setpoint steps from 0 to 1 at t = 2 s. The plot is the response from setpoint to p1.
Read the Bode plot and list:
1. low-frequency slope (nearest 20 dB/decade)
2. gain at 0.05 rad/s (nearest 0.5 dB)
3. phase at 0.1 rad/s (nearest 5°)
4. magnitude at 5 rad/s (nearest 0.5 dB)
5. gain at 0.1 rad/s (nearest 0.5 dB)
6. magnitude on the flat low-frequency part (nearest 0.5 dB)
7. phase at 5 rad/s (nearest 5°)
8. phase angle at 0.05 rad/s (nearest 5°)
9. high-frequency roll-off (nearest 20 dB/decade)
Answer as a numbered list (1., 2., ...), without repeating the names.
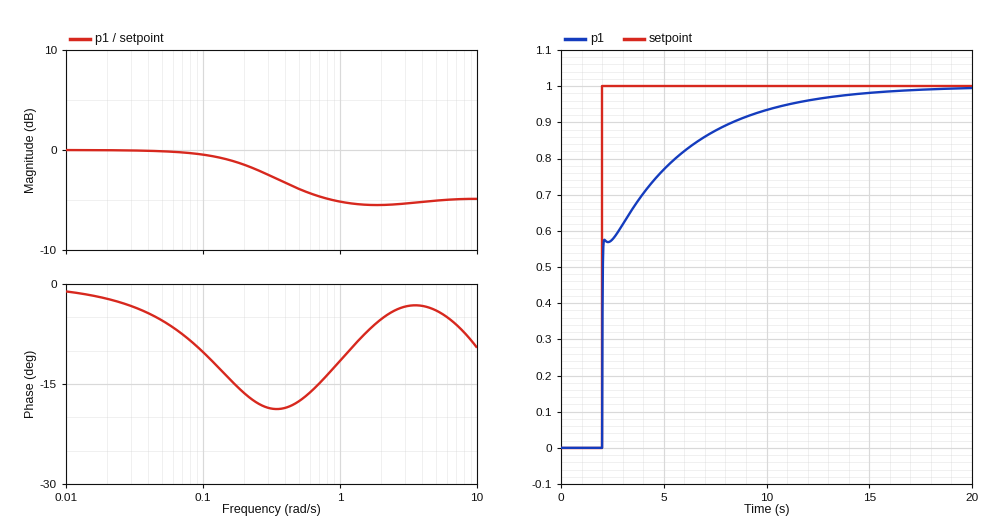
1. 0 dB/decade
2. 0.0 dB
3. -10°
4. -5.0 dB
5. -0.5 dB
6. 0.0 dB
7. -5°
8. -5°
9. 0 dB/decade
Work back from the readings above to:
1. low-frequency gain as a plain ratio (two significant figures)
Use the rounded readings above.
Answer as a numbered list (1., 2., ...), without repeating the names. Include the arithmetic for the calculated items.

1. 10^(0 / 20) = 1.0
